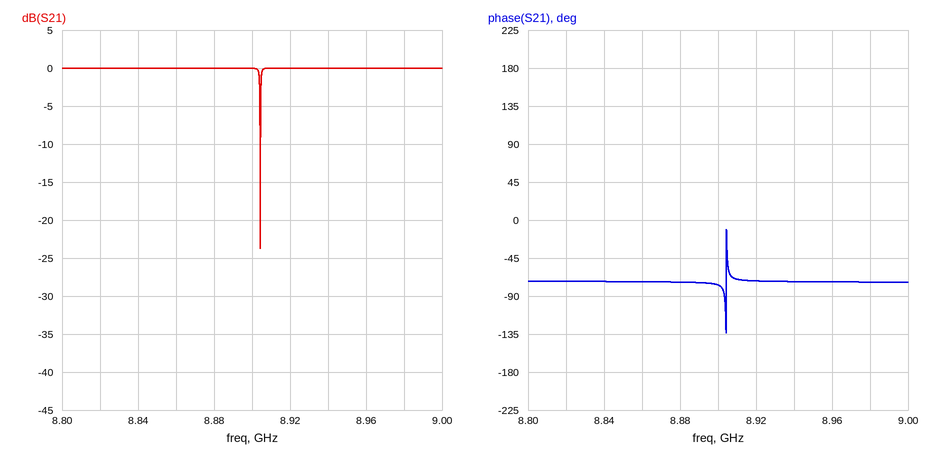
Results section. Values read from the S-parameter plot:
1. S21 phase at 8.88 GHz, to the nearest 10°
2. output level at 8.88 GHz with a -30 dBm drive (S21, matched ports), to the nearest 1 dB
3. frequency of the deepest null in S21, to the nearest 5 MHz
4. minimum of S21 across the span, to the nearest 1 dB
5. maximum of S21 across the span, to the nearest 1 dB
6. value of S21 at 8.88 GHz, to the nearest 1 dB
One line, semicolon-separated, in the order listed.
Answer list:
-70°; -30 dBm; 8.905 GHz; -24 dB; 0 dB; 0 dB
